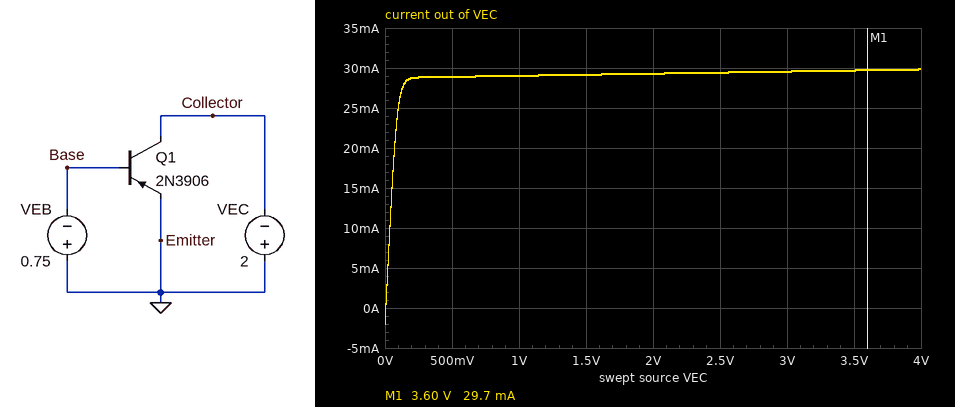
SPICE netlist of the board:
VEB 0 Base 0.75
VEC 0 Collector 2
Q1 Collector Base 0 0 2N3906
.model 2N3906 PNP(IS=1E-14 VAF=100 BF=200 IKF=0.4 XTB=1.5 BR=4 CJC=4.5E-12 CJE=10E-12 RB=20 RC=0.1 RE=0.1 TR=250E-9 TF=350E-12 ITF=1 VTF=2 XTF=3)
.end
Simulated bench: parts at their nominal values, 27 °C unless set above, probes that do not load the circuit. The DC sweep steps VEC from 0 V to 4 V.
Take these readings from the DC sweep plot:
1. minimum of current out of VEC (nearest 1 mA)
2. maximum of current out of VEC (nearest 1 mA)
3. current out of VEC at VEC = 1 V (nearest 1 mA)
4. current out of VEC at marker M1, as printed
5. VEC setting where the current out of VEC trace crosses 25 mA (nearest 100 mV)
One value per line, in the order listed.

-2 mA
30 mA
29 mA
29.7 mA
100 mV
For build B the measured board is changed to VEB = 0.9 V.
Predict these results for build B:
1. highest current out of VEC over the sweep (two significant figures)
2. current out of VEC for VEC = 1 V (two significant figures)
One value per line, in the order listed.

310 mA
300 mA
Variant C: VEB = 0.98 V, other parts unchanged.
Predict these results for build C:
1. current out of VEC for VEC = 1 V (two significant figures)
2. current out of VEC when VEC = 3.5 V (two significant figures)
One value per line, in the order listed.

460 mA
470 mA
